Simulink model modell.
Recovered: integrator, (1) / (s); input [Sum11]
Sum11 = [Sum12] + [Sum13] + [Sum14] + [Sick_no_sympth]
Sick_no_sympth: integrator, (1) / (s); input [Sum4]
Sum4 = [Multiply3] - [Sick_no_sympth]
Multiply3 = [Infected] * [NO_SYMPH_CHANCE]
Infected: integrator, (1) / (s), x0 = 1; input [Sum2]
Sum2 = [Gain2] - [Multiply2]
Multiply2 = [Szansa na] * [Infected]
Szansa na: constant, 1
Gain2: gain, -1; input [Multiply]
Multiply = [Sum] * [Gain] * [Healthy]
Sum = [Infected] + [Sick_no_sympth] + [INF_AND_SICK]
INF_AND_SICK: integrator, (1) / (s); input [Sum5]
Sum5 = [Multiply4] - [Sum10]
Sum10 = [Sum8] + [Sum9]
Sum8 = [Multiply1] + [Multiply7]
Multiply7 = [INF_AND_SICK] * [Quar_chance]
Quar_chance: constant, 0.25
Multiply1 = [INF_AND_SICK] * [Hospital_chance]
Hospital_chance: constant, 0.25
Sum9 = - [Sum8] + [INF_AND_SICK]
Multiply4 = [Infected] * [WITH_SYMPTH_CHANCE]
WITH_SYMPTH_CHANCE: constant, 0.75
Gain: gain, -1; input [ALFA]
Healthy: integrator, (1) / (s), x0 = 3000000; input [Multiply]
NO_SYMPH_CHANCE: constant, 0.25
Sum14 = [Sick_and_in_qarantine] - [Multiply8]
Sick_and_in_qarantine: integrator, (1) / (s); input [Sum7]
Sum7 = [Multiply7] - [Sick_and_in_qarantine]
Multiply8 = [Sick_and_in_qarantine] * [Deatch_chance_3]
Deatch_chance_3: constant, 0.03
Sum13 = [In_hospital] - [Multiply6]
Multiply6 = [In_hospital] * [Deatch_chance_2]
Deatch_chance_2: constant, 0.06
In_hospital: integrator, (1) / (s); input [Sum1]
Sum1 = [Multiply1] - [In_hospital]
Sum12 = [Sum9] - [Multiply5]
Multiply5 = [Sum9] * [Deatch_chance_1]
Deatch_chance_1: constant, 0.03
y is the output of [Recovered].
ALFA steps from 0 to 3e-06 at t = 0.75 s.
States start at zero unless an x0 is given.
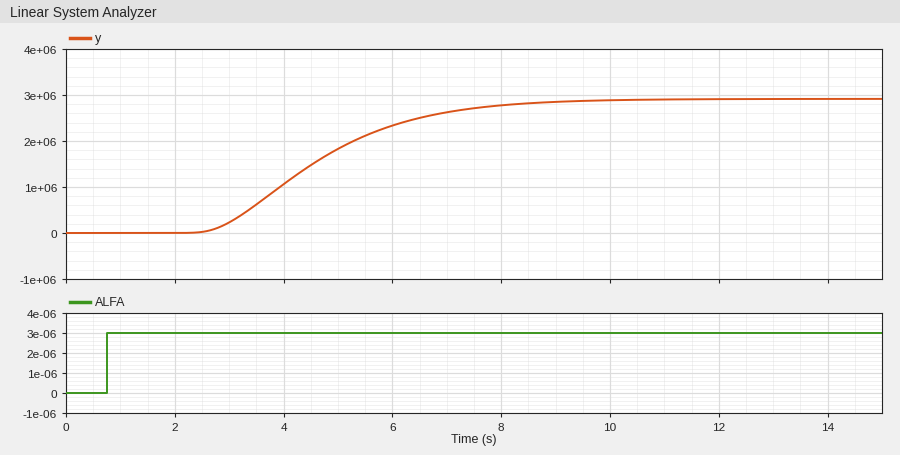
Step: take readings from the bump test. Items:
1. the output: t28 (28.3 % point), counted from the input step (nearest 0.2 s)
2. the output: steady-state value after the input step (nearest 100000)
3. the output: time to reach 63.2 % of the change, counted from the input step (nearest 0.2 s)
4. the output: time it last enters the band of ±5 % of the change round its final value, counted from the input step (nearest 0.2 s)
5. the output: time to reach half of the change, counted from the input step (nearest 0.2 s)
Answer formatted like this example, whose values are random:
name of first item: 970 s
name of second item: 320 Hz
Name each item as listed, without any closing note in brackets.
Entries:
the output: t28 (28.3 % point), counted from the input step: 3.0 s
the output: steady-state value after the input step: 2900000
the output: time to reach 63.2 % of the change, counted from the input step: 4.2 s
the output: time it last enters the band of ±5 % of the change round its final value, counted from the input step: 7.2 s
the output: time to reach half of the change, counted from the input step: 3.8 s
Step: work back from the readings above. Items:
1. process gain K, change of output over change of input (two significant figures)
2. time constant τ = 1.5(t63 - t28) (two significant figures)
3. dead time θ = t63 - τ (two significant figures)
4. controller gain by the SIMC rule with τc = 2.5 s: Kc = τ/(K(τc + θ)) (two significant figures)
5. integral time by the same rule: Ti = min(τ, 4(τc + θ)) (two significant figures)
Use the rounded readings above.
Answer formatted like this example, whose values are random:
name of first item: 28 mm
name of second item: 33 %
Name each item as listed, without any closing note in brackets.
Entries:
process gain K, change of output over change of input: 970000000000
time constant τ = 1.5(t63 - t28): 1.8 s
dead time θ = t63 - τ: 2.4 s
controller gain by the SIMC rule with τc = 2.5 s: Kc = τ/(K(τc + θ)): 0.00000000000038
integral time by the same rule: Ti = min(τ, 4(τc + θ)): 1.8 s
